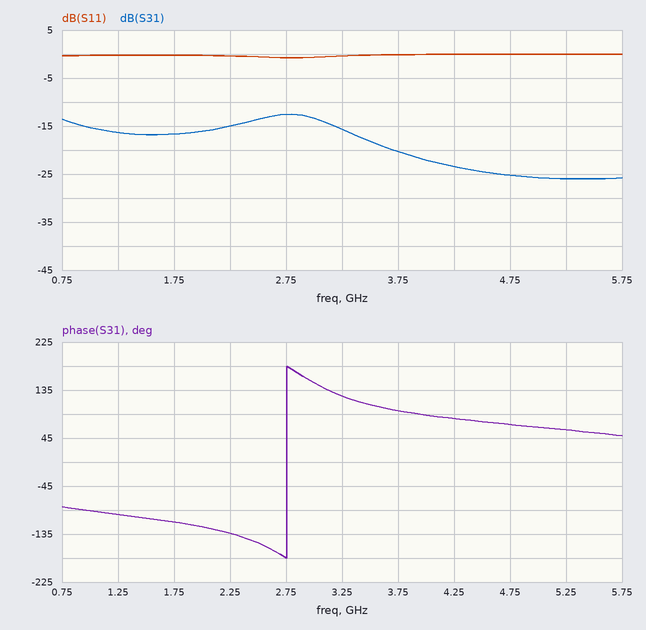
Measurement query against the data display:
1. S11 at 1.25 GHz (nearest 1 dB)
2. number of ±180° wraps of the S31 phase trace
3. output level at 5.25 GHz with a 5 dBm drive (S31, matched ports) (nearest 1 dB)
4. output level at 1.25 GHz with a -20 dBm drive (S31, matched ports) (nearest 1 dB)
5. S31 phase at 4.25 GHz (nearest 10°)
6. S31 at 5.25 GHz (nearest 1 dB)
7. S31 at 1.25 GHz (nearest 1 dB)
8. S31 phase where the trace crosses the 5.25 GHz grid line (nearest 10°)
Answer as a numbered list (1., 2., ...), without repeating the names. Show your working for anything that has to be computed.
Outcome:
1. 0 dB
2. 1
3. 5 dBm + (-26 dB) = -21 dBm
4. -20 dBm + (-16 dB) = -36 dBm
5. 80°
6. -26 dB
7. -16 dB
8. 60°
